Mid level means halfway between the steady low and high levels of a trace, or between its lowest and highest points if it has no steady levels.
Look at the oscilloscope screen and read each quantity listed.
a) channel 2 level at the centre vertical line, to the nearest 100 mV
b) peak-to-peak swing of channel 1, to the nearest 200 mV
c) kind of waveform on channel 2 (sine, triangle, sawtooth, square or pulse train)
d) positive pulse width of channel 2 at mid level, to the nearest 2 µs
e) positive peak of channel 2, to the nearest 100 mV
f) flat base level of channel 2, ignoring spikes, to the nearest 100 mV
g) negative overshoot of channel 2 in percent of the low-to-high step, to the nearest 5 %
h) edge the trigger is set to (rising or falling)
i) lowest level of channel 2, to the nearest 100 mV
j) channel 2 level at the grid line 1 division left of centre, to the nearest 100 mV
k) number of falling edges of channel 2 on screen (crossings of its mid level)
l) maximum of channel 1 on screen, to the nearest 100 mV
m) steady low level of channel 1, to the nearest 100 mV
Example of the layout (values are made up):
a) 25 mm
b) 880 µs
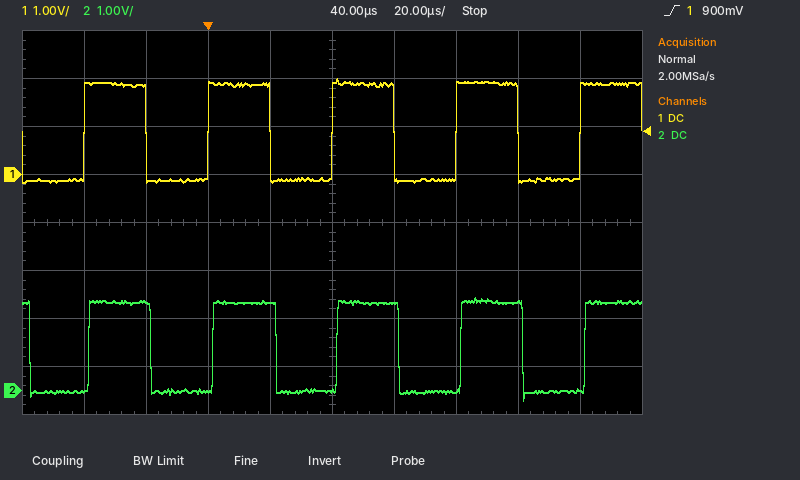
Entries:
a) 0.0 V
b) 2.2 V
c) square
d) 20 µs
e) 1.9 V
f) 0.0 V
g) 10 %
h) rising
i) -200 mV
j) 1.8 V
k) 5
l) 2.0 V
m) -100 mV
